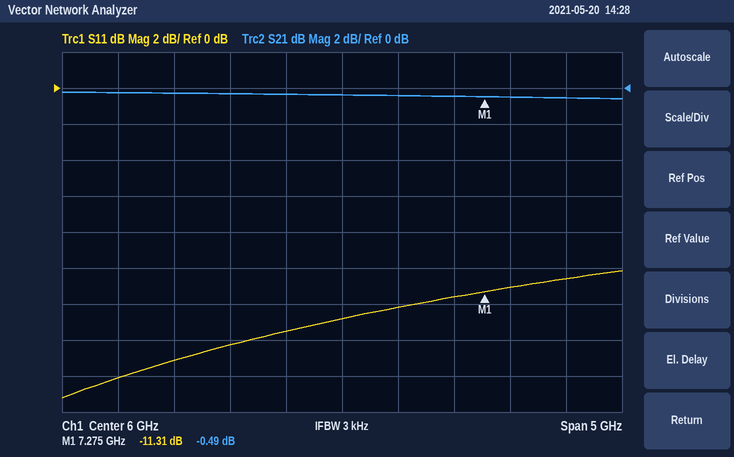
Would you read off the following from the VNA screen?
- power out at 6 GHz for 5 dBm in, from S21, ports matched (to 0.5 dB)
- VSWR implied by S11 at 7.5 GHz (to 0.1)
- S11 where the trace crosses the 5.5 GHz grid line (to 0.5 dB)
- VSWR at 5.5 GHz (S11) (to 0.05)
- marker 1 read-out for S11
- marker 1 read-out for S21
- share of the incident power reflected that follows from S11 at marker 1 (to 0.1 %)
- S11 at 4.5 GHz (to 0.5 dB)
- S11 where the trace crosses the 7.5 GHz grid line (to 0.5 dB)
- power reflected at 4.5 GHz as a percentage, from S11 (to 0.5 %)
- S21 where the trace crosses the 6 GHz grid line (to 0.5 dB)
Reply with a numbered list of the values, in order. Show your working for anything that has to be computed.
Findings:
1. 5 dBm + (-0.5 dB) = 4.5 dBm
2. |Γ| = 10^(-11/20) = 0.2818; VSWR = (1 + 0.2818)/(1 − 0.2818) ≈ 1.8
3. -13.5 dB
4. |Γ| = 10^(-13.5/20) = 0.2113; VSWR = (1 + 0.2113)/(1 − 0.2113) ≈ 1.54, so 1.55 to the nearest 0.05
5. -11.31 dB
6. -0.49 dB
7. 10^(-11.31/10) ≈ 7.4 %
8. -15.0 dB
9. -11.0 dB
10. 10^(-15/10) ≈ 3.16 %, so 3.0 % to the nearest 0.5 %
11. -0.5 dB
